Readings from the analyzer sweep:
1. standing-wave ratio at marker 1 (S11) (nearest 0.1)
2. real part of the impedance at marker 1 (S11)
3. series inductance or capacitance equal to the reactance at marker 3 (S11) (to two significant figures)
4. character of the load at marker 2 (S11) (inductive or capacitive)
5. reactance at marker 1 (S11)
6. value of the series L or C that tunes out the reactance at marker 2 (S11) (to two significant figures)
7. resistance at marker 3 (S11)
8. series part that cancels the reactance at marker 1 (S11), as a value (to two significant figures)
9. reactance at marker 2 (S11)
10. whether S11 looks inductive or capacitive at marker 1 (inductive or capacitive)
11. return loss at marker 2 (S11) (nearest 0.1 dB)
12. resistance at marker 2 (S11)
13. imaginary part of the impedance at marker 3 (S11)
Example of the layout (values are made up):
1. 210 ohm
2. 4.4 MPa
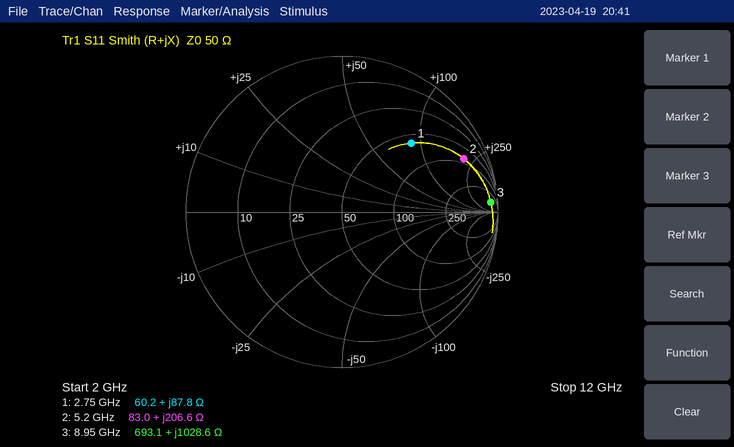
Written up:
1. 4.4
2. 60.2 Ω
3. 18 nH
4. inductive
5. +87.8 Ω
6. 150 fF
7. 693.1 Ω
8. 660 fF
9. +206.6 Ω
10. inductive
11. 1.4 dB
12. 83.0 Ω
13. +1028.6 Ω
